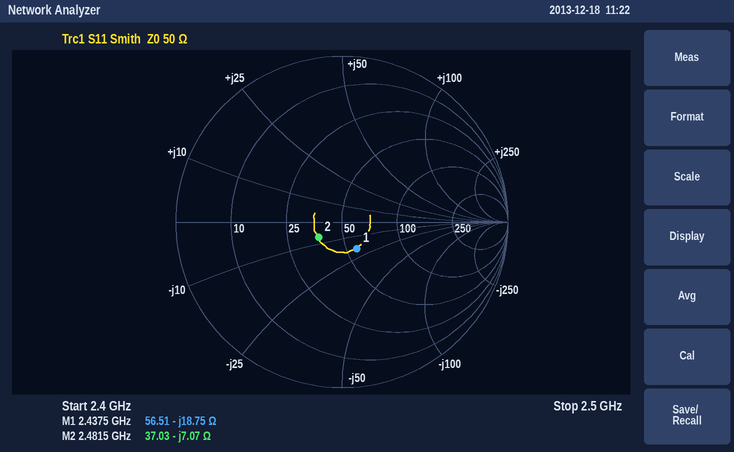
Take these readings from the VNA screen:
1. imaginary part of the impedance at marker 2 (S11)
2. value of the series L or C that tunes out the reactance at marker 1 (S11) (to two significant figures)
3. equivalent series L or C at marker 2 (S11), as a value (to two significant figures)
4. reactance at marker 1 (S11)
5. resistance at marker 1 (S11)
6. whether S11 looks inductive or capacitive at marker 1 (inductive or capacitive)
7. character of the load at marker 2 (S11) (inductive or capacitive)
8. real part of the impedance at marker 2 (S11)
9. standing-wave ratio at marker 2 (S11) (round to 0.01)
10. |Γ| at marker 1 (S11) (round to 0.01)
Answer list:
-7.07 Ω
1.2 nH
9.1 pF
-18.75 Ω
56.51 Ω
capacitive
capacitive
37.03 Ω
1.41
0.18
